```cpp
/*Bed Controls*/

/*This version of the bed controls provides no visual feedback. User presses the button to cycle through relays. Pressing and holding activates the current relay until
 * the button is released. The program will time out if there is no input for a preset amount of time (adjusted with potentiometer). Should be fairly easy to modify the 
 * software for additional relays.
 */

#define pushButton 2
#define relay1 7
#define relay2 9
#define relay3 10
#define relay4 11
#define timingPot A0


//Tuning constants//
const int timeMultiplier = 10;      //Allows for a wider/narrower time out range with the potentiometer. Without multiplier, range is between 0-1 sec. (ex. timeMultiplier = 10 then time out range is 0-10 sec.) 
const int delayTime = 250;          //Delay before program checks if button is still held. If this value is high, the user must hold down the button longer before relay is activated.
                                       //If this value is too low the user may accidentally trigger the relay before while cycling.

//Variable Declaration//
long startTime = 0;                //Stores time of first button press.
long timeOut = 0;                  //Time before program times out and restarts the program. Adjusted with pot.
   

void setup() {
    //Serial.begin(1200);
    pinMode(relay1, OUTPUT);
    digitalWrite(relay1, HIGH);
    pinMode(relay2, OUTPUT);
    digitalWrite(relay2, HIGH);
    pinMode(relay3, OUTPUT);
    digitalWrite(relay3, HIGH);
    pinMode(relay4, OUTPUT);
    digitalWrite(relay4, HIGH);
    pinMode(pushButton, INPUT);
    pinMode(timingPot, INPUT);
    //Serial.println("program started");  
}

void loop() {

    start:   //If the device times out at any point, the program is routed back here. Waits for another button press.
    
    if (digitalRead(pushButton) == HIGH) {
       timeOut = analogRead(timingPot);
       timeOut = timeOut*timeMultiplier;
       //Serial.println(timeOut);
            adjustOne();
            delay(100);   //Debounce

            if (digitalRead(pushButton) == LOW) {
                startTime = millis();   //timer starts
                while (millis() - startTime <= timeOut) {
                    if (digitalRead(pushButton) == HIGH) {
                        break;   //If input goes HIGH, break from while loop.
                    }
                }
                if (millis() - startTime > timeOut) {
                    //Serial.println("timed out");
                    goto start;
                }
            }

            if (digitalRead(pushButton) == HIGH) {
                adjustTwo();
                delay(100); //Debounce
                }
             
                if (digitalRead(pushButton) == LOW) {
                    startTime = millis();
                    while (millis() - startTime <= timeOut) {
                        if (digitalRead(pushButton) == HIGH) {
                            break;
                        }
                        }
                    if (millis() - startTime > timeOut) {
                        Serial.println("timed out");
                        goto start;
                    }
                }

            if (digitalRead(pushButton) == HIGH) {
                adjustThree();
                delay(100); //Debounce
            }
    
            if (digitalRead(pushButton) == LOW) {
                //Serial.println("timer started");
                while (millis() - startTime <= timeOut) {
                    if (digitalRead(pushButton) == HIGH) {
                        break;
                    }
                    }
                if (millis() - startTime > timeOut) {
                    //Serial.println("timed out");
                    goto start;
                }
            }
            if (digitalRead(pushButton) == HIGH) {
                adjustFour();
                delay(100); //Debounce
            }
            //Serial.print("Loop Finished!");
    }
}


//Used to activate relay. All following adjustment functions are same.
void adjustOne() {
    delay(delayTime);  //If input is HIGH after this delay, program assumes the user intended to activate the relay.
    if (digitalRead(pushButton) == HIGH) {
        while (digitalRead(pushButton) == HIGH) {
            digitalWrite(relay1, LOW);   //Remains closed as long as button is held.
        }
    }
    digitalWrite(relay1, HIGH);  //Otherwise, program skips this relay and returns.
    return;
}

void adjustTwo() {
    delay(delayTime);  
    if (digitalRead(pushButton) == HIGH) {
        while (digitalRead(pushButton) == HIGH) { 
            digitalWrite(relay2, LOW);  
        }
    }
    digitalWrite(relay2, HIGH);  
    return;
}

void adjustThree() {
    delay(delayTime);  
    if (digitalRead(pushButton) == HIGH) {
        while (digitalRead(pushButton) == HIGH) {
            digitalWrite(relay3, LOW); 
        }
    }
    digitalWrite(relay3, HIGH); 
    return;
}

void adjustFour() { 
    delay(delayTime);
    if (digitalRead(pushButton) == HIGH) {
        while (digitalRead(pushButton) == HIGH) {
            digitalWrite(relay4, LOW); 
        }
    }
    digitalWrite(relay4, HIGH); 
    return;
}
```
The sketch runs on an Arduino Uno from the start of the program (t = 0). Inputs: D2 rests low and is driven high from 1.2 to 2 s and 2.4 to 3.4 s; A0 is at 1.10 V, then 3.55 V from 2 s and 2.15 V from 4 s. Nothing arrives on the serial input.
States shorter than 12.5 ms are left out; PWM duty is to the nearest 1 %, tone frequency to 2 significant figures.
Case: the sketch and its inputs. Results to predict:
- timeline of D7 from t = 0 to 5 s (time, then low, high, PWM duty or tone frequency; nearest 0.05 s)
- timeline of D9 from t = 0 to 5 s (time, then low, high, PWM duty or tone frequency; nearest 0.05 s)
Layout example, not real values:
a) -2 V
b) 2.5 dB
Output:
a) 0 s high; 1.45 s low; 2 s high
b) 0 s high; 2.65 s low; 3.4 s high
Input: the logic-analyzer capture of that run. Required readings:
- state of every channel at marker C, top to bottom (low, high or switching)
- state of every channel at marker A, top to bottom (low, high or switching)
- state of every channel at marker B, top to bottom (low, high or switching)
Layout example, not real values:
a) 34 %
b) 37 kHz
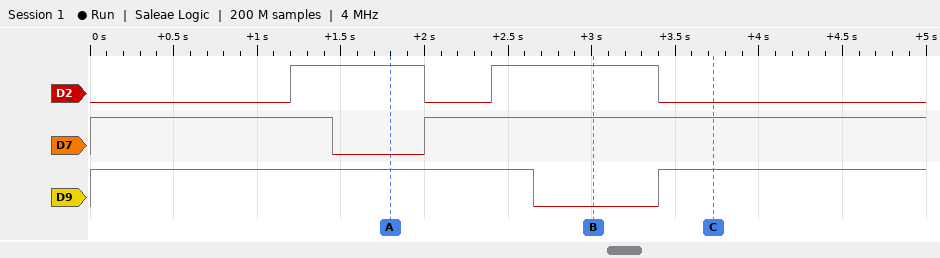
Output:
a) D2 low, D7 high, D9 high
b) D2 high, D7 low, D9 high
c) D2 high, D7 high, D9 low
